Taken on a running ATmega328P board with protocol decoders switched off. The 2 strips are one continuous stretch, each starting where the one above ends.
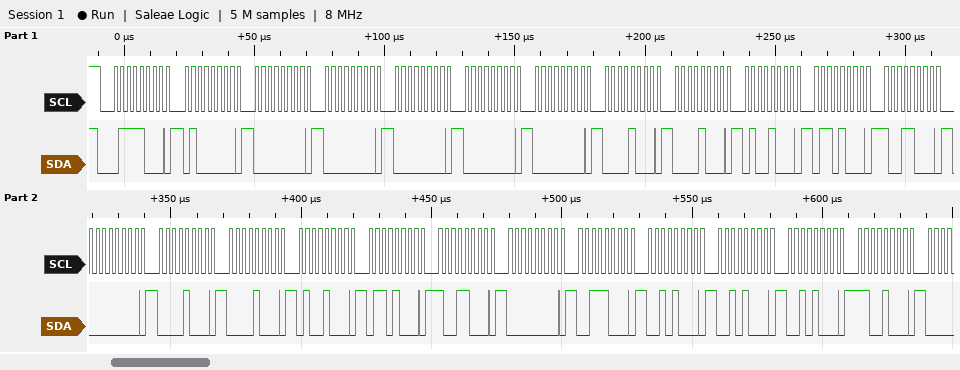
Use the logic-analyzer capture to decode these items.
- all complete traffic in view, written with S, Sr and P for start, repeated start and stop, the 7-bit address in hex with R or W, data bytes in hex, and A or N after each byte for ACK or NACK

S 3CW A 40 A 00 A 00 A 00 A 00 A 00 A 08 A 08 A 48 A 68 A 98 A 00 A 08 A 08 A 48 A 68 A 98 A 00 A 38 A 28 A 28 A 28 A C8 A
